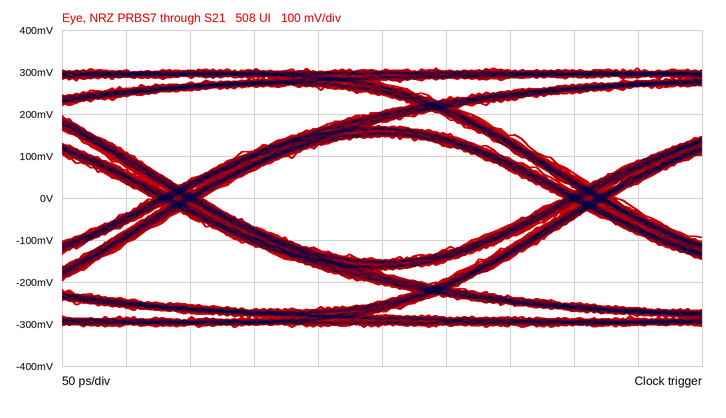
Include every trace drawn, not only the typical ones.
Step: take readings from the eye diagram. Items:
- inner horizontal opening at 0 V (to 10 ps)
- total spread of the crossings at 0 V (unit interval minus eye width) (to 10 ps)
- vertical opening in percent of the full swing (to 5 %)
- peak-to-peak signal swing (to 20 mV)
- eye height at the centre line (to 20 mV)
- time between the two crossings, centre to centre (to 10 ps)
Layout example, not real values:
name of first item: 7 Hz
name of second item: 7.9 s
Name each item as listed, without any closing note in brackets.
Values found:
inner horizontal opening at 0 V: 280 ps
total spread of the crossings at 0 V (unit interval minus eye width): 40 ps
vertical opening in percent of the full swing: 50 %
peak-to-peak signal swing: 620 mV
eye height at the centre line: 300 mV
time between the two crossings, centre to centre: 320 ps
